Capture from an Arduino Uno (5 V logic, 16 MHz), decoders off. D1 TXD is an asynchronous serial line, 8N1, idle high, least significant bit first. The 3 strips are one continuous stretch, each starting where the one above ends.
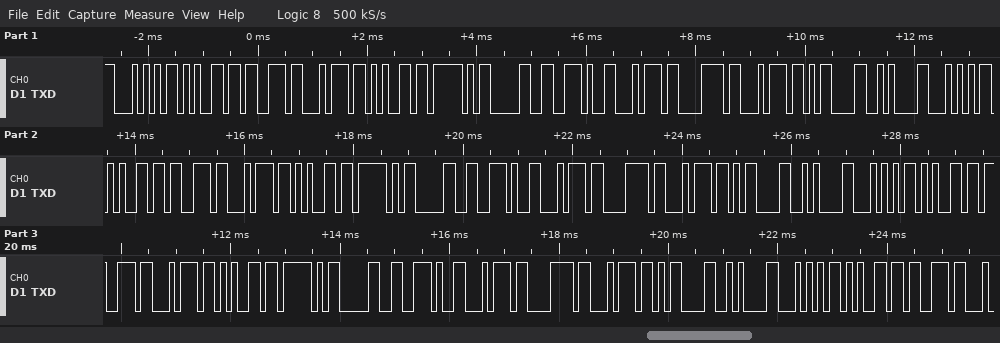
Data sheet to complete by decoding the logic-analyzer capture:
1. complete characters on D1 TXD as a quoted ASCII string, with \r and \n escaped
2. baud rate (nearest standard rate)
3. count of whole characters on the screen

"Teste_0.txt\r\nTeste_0.txt\r\nTeste_0.txt\r\nTes"
9600 baud
42
